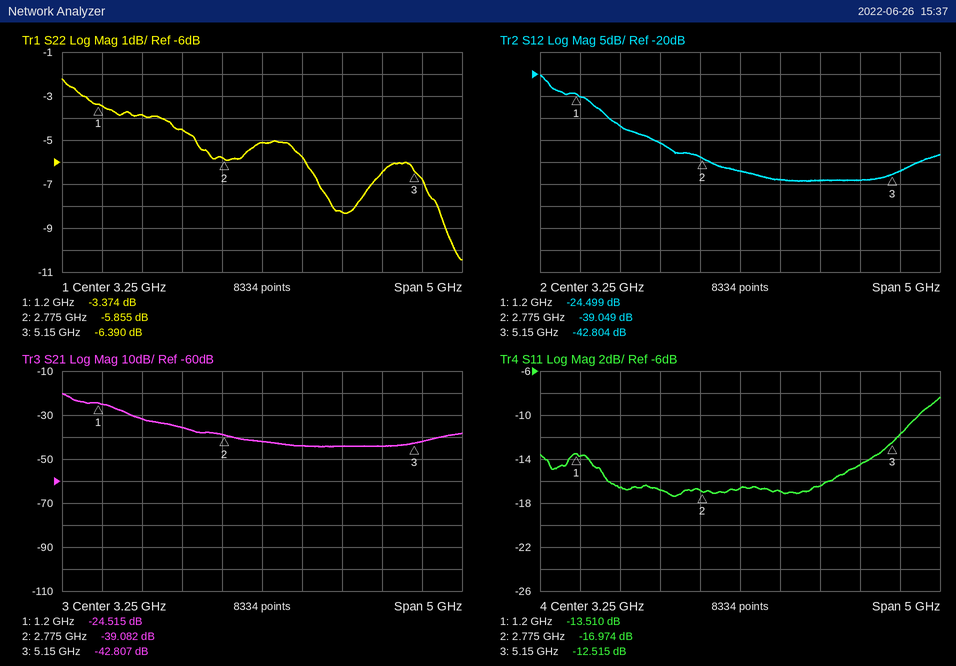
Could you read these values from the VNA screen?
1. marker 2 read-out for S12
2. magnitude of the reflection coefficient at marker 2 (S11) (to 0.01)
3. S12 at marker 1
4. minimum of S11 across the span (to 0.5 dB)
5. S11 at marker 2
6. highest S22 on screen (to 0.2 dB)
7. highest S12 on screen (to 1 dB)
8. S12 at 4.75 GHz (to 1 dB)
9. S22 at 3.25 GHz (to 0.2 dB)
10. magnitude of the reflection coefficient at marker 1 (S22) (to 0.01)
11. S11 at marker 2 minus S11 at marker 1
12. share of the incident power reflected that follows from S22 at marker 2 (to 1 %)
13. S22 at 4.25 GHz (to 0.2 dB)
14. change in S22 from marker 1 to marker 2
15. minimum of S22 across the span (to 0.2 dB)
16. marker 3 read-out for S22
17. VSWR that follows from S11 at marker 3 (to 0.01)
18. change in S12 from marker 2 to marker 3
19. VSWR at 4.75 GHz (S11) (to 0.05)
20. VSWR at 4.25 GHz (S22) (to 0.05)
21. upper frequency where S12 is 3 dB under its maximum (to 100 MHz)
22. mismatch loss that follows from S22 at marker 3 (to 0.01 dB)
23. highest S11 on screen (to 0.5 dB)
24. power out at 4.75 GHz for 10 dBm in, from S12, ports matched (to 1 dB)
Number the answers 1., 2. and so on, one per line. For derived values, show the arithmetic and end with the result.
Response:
1. -39.049 dB
2. 10^(-16.974/20) ≈ 0.14
3. -24.499 dB
4. -17.5 dB
5. -16.974 dB
6. -2.2 dB
7. -20 dB
8. -44 dB
9. -5.2 dB
10. 10^(-3.374/20) ≈ 0.68
11. -16.974 − (-13.51) = -3.464 dB
12. 10^(-5.855/10) ≈ 26 %
13. -8.2 dB
14. -5.855 − (-3.374) = -2.481 dB
15. -10.4 dB
16. -6.390 dB
17. (1 + 0.2367)/(1 − 0.2367) ≈ 1.62
18. -42.804 − (-39.049) = -3.755 dB
19. |Γ| = 10^(-14.5/20) = 0.1884; VSWR = (1 + 0.1884)/(1 − 0.1884) ≈ 1.46, so 1.45 to the nearest 0.05
20. |Γ| = 10^(-8.2/20) = 0.3890; VSWR = (1 + 0.3890)/(1 − 0.3890) ≈ 2.27, so 2.25 to the nearest 0.05
21. 900 MHz
22. −10 log10(1 − 10^(-6.39/10)) ≈ 1.13 dB
23. -8.5 dB
24. 10 dBm + (-44 dB) = -34 dBm
